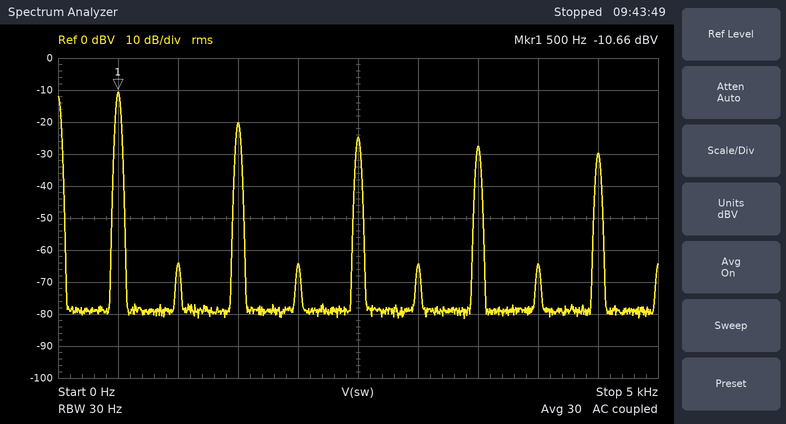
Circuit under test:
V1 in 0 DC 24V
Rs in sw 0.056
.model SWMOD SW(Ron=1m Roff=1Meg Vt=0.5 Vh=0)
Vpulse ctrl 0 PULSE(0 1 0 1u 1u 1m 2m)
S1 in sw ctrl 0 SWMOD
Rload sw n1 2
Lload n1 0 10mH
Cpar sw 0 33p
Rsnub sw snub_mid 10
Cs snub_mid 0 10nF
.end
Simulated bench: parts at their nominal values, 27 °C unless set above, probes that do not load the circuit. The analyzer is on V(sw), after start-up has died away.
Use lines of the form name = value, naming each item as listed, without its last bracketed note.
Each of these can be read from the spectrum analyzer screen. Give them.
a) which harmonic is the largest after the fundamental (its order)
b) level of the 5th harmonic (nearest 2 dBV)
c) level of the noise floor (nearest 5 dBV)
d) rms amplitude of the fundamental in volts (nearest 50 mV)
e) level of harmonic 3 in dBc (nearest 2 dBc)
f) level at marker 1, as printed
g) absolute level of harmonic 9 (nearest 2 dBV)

which harmonic is the largest after the fundamental = 3
level of the 5th harmonic = -24 dBV
level of the noise floor = -80 dBV
rms amplitude of the fundamental in volts = 300 mV
level of harmonic 3 in dBc = -10 dBc
level at marker 1, as printed = -10.66 dBV
absolute level of harmonic 9 = -30 dBV
